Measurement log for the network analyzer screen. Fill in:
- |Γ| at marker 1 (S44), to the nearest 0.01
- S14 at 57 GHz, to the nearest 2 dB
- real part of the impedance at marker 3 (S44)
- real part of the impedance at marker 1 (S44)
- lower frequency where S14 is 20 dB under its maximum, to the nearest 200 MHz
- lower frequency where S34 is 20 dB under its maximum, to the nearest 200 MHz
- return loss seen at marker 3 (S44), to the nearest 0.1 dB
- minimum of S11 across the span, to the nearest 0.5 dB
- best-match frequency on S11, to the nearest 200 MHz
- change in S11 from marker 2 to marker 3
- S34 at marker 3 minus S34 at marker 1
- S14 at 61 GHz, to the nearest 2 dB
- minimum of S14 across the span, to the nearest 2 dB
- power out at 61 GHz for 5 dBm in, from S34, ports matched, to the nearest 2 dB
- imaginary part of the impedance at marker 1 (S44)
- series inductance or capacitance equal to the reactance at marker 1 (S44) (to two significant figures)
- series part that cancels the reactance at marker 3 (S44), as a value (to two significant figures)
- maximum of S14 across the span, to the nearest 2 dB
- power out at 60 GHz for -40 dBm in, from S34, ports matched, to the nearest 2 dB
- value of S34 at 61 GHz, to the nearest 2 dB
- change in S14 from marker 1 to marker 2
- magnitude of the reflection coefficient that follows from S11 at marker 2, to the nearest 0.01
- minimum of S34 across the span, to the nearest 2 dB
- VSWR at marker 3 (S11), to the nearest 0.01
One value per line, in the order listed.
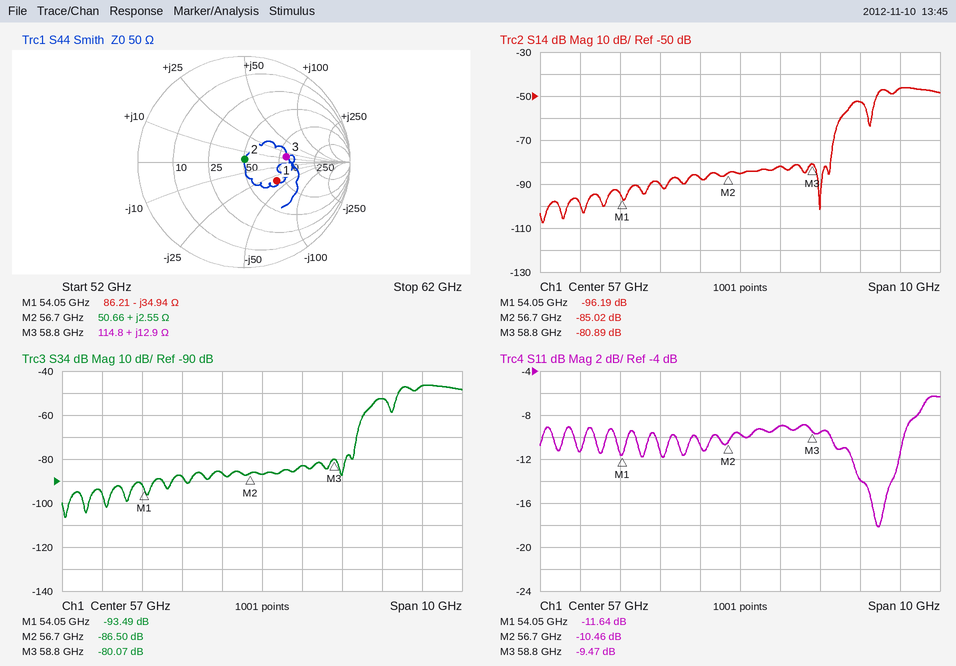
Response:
0.36
-86 dB
114.8 Ω
86.21 Ω
59.4 GHz
59.4 GHz
8.0 dB
-18.0 dB
60.4 GHz
0.99 dB
13.42 dB
-46 dB
-108 dB
-42 dBm
-34.94 Ω
84 fF
210 fF
-46 dB
-92 dBm
-46 dB
11.17 dB
0.30
-106 dB
2.01
